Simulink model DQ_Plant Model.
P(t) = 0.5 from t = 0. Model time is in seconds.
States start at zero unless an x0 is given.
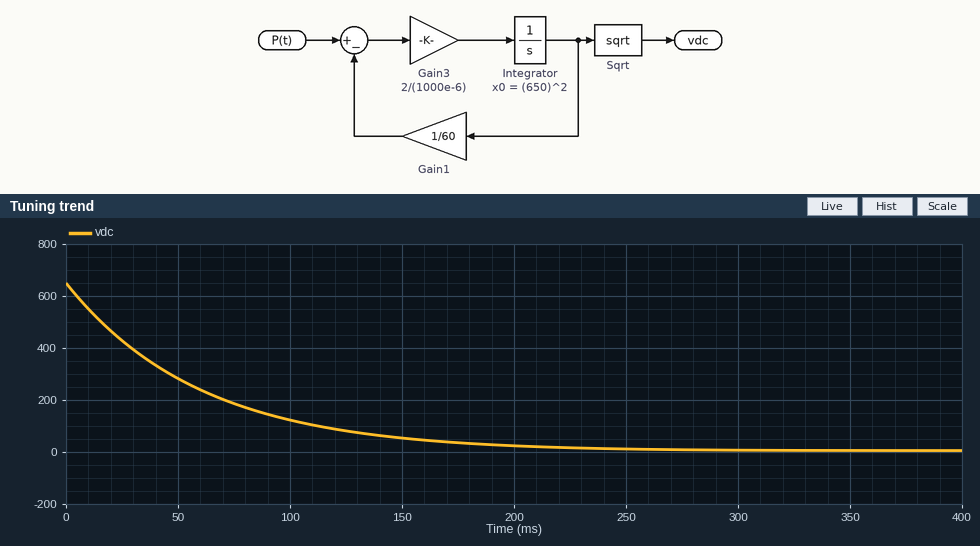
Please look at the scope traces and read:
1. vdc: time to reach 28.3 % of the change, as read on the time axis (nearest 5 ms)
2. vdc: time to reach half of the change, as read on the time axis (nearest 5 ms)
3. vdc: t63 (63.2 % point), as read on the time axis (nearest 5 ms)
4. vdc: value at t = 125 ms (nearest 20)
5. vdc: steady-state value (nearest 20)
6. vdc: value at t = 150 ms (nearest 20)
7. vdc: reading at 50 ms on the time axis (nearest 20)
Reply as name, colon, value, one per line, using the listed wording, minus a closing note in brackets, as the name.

vdc: time to reach 28.3 % of the change, as read on the time axis: 20 ms
vdc: time to reach half of the change, as read on the time axis: 40 ms
vdc: t63 (63.2 % point), as read on the time axis: 60 ms
vdc: value at t = 125 ms: 80
vdc: steady-state value: 0
vdc: value at t = 150 ms: 60
vdc: reading at 50 ms on the time axis: 280
